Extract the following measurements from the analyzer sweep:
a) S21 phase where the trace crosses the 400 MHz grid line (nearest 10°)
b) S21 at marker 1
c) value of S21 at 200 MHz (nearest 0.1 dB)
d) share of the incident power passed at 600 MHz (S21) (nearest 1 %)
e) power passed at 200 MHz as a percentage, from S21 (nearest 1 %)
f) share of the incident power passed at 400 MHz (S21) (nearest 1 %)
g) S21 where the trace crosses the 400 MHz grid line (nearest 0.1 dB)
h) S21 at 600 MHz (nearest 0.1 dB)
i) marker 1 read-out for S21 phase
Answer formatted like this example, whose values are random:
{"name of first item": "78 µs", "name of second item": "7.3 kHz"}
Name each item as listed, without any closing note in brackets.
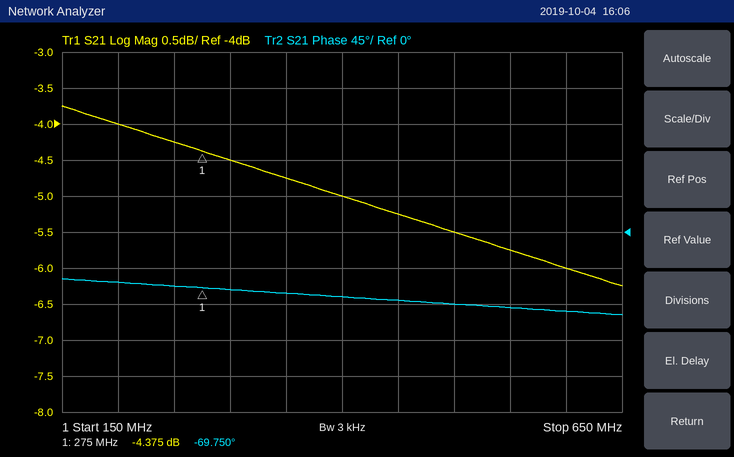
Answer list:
{"S21 phase where the trace crosses the 400 MHz grid line": "-80°", "S21 at marker 1": "-4.375 dB", "value of S21 at 200 MHz": "-4.0 dB", "share of the incident power passed at 600 MHz (S21)": "25 %", "power passed at 200 MHz as a percentage, from S21": "40 %", "share of the incident power passed at 400 MHz (S21)": "32 %", "S21 where the trace crosses the 400 MHz grid line": "-5.0 dB", "S21 at 600 MHz": "-6.0 dB", "marker 1 read-out for S21 phase": "-69.750°"}
